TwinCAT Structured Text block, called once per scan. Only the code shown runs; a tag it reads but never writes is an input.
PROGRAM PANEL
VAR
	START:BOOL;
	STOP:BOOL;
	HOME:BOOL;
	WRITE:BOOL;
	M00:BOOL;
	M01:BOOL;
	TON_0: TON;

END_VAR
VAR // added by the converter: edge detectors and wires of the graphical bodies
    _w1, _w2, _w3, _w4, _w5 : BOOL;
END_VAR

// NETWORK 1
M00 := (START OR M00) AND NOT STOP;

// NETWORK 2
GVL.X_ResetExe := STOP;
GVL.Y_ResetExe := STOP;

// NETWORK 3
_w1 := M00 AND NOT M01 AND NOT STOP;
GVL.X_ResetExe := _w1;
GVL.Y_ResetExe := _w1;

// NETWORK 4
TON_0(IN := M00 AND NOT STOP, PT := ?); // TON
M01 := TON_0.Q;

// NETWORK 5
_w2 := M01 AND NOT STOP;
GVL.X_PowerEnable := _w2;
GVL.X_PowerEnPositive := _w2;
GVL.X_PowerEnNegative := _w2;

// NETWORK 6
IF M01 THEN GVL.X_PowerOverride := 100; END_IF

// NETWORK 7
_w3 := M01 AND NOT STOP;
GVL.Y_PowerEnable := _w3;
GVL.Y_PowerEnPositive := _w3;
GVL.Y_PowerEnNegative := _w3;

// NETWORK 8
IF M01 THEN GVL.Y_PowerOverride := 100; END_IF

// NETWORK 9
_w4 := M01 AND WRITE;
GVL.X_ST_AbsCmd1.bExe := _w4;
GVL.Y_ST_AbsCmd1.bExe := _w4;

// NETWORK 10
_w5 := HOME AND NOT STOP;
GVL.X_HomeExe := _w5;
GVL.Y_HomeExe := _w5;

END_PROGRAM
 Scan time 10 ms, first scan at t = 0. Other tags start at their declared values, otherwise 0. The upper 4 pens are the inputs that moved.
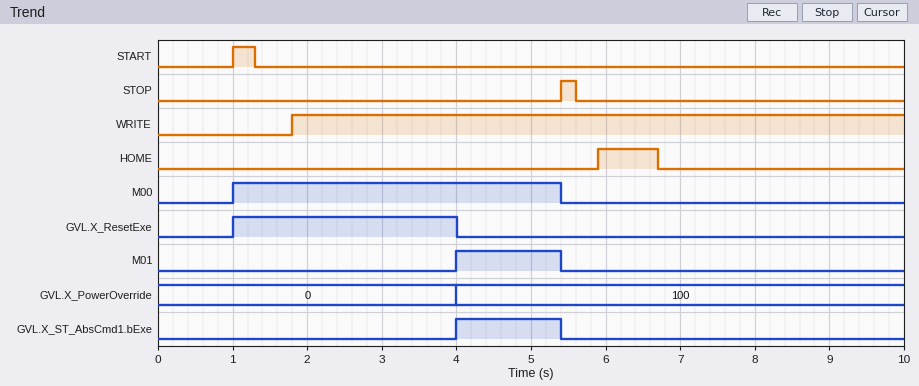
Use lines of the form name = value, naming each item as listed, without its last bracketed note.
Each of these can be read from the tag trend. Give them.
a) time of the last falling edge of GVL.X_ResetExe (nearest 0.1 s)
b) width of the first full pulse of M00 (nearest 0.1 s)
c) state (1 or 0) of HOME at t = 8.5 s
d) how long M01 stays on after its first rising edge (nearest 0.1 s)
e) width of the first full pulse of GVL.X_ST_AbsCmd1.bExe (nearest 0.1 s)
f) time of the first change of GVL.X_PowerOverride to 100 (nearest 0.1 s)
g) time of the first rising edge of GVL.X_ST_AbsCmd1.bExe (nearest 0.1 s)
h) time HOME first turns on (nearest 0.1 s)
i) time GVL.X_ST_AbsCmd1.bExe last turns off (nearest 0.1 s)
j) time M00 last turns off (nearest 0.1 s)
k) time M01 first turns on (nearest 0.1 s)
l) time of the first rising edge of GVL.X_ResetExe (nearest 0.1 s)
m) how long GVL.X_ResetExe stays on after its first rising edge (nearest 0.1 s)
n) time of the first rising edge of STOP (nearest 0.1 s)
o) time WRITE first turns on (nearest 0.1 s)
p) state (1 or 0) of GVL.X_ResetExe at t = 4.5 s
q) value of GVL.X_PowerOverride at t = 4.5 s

time of the last falling edge of GVL.X_ResetExe = 4.0 s
width of the first full pulse of M00 = 4.4 s
state (1 or 0) of HOME at t = 8.5 s = 0
how long M01 stays on after its first rising edge = 1.4 s
width of the first full pulse of GVL.X_ST_AbsCmd1.bExe = 1.4 s
time of the first change of GVL.X_PowerOverride to 100 = 4.0 s
time of the first rising edge of GVL.X_ST_AbsCmd1.bExe = 4.0 s
time HOME first turns on = 5.9 s
time GVL.X_ST_AbsCmd1.bExe last turns off = 5.4 s
time M00 last turns off = 5.4 s
time M01 first turns on = 4.0 s
time of the first rising edge of GVL.X_ResetExe = 1.0 s
how long GVL.X_ResetExe stays on after its first rising edge = 3.0 s
time of the first rising edge of STOP = 5.4 s
time WRITE first turns on = 1.8 s
state (1 or 0) of GVL.X_ResetExe at t = 4.5 s = 0
value of GVL.X_PowerOverride at t = 4.5 s = 100
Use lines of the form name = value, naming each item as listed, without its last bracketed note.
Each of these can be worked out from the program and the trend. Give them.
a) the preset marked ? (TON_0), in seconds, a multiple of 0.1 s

the preset marked ? (TON_0), in seconds, a multiple of 0.1 s = 3.0 s
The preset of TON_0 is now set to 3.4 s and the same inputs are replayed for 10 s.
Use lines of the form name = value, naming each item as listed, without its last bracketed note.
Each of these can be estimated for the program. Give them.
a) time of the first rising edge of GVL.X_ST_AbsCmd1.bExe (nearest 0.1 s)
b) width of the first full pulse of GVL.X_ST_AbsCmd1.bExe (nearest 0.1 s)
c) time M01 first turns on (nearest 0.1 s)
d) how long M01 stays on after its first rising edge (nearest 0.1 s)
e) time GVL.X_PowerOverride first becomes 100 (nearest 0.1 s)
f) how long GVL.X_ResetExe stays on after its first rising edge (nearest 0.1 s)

time of the first rising edge of GVL.X_ST_AbsCmd1.bExe = 4.4 s
width of the first full pulse of GVL.X_ST_AbsCmd1.bExe = 1.0 s
time M01 first turns on = 4.4 s
how long M01 stays on after its first rising edge = 1.0 s
time GVL.X_PowerOverride first becomes 100 = 4.4 s
how long GVL.X_ResetExe stays on after its first rising edge = 3.4 s
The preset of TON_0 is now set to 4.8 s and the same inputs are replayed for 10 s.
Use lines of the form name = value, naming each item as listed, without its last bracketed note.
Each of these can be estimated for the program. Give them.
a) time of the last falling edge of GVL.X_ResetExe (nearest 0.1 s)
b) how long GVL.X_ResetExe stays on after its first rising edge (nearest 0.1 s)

time of the last falling edge of GVL.X_ResetExe = 5.4 s
how long GVL.X_ResetExe stays on after its first rising edge = 4.4 s
